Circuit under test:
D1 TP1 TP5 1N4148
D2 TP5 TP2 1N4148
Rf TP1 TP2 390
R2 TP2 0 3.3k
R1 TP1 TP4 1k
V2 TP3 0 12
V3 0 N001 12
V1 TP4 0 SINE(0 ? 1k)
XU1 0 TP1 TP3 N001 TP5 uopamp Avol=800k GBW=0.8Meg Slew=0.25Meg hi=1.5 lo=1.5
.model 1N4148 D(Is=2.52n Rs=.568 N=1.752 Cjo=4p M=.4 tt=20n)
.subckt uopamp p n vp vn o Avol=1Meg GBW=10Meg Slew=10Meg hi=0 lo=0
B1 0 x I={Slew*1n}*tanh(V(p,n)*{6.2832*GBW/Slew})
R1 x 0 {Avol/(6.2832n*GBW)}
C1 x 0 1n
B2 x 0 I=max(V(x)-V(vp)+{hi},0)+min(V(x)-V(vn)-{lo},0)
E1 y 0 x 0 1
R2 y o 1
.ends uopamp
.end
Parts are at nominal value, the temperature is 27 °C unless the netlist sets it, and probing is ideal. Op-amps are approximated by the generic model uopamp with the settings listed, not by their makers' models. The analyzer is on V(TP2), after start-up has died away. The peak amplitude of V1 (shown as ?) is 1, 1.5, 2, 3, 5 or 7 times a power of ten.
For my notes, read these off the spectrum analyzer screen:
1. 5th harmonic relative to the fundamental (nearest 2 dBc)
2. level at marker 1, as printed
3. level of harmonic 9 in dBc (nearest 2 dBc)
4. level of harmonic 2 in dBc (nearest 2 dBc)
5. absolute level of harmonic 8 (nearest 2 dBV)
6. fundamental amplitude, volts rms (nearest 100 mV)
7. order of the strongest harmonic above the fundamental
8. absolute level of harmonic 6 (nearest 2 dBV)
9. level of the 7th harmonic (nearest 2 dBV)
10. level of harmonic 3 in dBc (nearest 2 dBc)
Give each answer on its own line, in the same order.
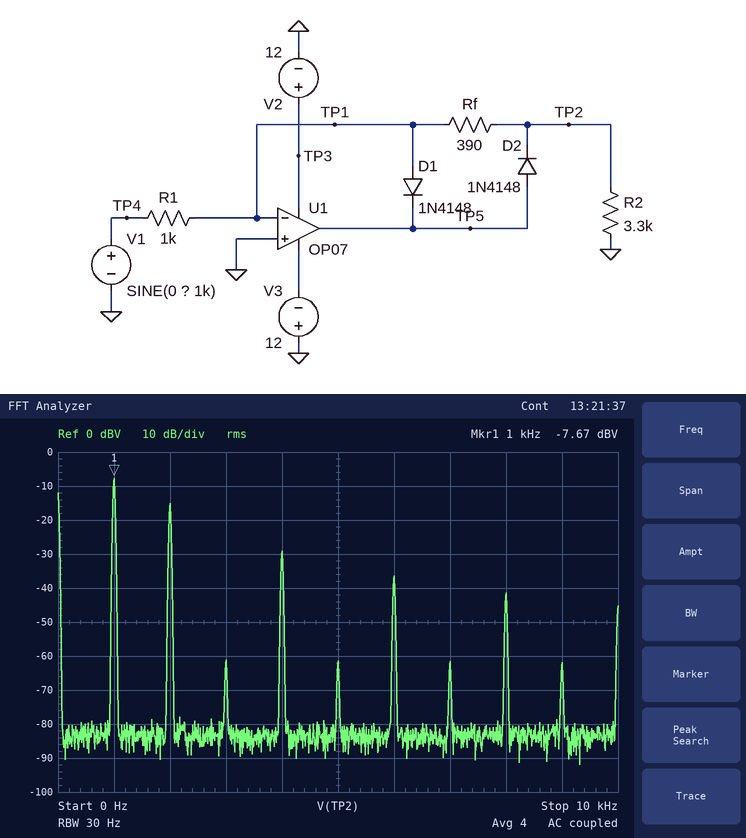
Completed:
-54 dBc
-7.67 dBV
-54 dBc
-8 dBc
-42 dBV
400 mV
2
-36 dBV
-62 dBV
-54 dBc
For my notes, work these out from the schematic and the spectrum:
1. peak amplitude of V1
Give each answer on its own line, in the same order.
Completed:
3 V
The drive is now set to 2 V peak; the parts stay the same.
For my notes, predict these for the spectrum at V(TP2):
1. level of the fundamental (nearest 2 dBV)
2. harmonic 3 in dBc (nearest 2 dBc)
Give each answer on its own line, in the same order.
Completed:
-12 dBV
-50 dBc
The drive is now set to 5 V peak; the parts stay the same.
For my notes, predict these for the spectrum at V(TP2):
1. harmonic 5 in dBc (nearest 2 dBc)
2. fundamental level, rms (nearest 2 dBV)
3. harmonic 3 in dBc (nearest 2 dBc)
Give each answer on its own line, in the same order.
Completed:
-56 dBc
-4 dBV
-56 dBc
